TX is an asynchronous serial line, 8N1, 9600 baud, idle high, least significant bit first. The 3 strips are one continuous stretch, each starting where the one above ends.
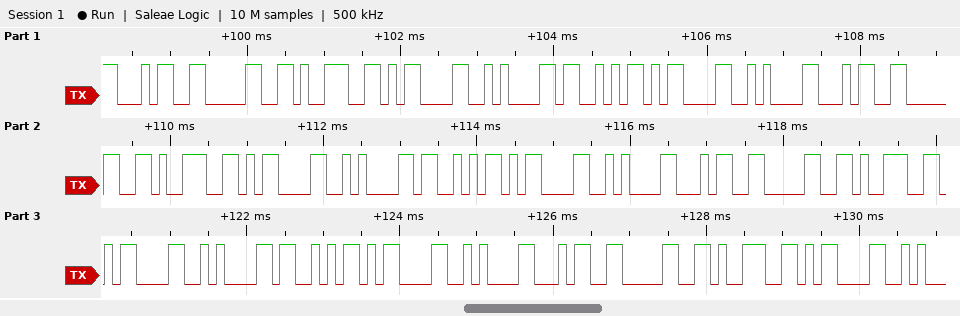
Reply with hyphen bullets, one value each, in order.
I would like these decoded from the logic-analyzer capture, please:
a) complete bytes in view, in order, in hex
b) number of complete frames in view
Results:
- 0x34 0x30 0x39 0x0D 0x0A 0x53 0x0D 0x0A 0x34 0x30 0x39 0x0D 0x0A 0x53 0x0D 0x0A 0x34 0x30 0x39 0x0D 0x0A 0x53 0x0D 0x0A 0x34 0x30 0x39 0x0D
- 28
